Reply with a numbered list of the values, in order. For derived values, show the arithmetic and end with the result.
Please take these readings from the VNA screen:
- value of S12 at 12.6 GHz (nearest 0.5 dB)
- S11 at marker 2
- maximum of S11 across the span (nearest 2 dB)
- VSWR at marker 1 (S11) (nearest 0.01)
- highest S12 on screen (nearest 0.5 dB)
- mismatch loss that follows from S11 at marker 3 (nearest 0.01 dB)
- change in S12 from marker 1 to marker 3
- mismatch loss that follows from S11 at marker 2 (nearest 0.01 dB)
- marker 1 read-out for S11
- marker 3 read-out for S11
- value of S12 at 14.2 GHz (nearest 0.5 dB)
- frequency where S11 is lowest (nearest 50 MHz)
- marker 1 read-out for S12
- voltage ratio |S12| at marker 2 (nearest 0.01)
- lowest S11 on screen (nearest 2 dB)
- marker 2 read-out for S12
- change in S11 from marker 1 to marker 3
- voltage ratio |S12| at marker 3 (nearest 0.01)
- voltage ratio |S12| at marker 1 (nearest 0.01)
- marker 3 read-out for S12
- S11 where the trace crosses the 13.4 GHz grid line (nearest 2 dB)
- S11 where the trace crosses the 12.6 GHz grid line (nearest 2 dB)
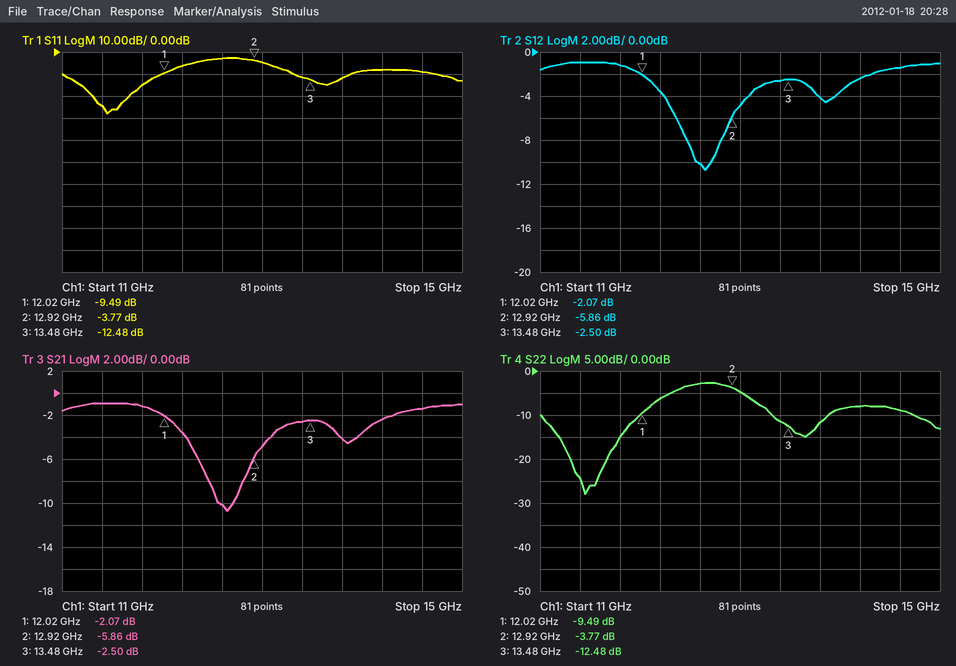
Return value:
1. -10.0 dB
2. -3.77 dB
3. -2 dB
4. (1 + 0.3354)/(1 − 0.3354) ≈ 2.01
5. -1.0 dB
6. −10 log10(1 − 10^(-12.48/10)) ≈ 0.25 dB
7. -2.5 − (-2.07) = -0.43 dB
8. −10 log10(1 − 10^(-3.77/10)) ≈ 2.36 dB
9. -9.49 dB
10. -12.48 dB
11. -2.5 dB
12. 11.45 GHz
13. -2.07 dB
14. 10^(-5.86/20) ≈ 0.51
15. -28 dB
16. -5.86 dB
17. -12.48 − (-9.49) = -2.99 dB
18. 10^(-2.5/20) ≈ 0.75
19. 10^(-2.07/20) ≈ 0.79
20. -2.50 dB
21. -12 dB
22. -2 dB
